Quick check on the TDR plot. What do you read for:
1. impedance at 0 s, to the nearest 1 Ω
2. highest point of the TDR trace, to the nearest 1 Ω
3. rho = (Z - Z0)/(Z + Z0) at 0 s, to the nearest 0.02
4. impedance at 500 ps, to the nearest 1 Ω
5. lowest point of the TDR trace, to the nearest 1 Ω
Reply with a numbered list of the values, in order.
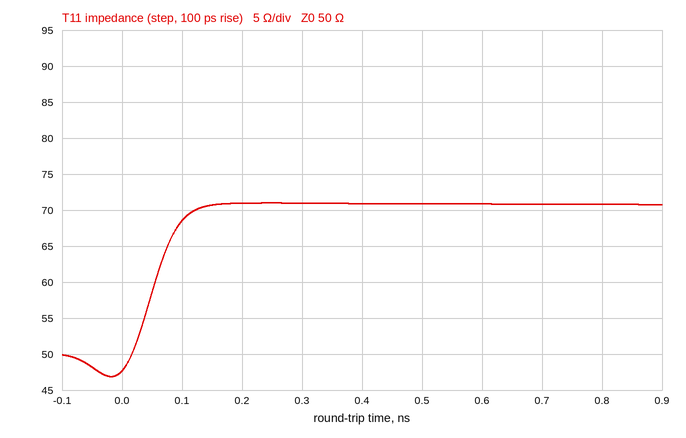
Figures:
1. 48 Ω
2. 71 Ω
3. -0.02
4. 71 Ω
5. 47 Ω
